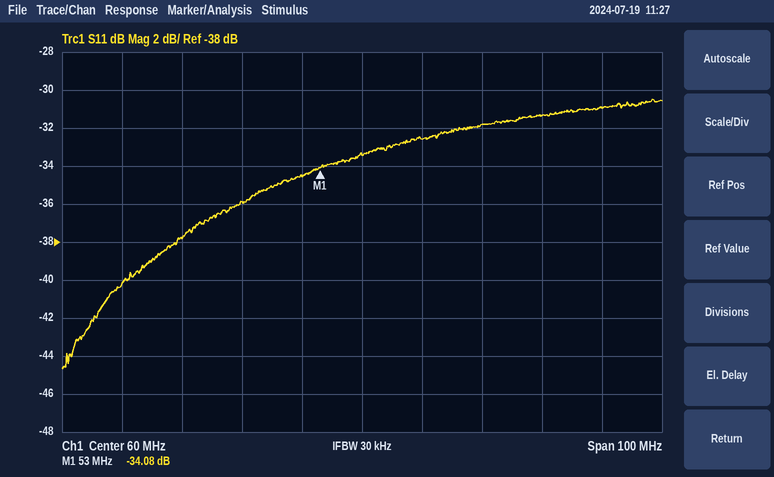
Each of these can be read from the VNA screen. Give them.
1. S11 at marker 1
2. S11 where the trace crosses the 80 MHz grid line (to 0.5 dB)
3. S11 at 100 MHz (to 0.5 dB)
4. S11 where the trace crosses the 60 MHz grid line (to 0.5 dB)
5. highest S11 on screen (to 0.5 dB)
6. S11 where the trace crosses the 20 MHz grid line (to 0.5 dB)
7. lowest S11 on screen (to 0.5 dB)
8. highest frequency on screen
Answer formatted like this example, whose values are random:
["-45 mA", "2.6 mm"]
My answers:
["-34.08 dB", "-32.0 dB", "-31.0 dB", "-33.5 dB", "-30.5 dB", "-40.0 dB", "-44.5 dB", "110 MHz"]
